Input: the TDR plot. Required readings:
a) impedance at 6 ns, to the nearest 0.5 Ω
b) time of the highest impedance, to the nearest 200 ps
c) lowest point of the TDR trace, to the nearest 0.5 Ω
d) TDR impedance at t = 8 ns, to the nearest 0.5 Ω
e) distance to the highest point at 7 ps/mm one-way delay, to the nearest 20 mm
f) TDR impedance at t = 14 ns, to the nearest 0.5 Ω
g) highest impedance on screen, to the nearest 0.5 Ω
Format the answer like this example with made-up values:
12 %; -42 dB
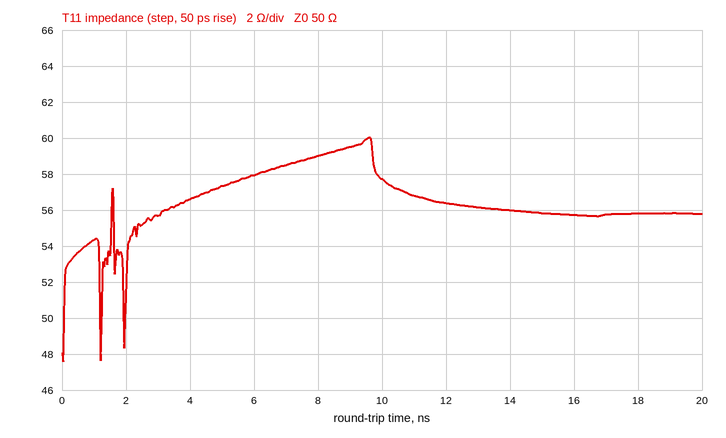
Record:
58.0 Ω; 9.6 ns; 47.5 Ω; 59.0 Ω; 680 mm; 56.0 Ω; 60.0 Ω
